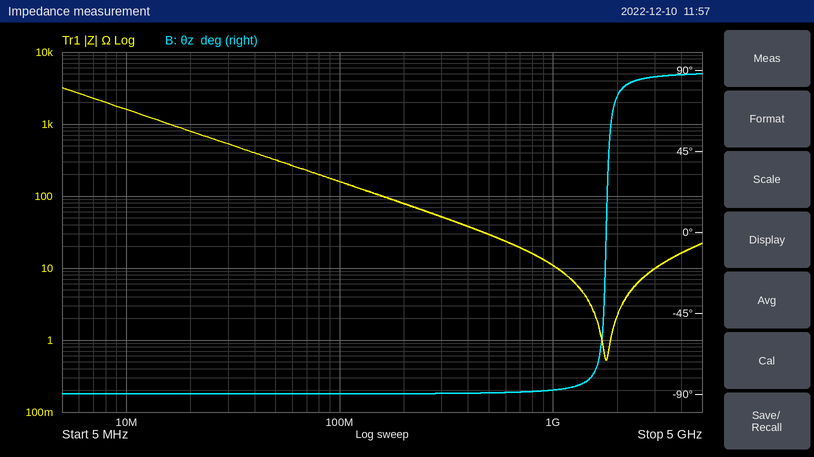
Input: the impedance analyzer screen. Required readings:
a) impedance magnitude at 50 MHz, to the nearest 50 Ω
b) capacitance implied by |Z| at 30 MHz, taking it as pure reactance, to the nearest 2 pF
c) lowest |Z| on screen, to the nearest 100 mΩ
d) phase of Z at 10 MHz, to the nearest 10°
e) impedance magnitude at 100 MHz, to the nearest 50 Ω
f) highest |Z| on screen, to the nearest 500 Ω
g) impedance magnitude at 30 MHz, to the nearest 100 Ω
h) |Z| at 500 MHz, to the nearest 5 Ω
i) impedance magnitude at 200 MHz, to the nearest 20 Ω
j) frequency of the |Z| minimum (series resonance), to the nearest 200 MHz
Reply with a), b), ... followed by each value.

a) 300 Ω
b) 10 pF
c) 500 mΩ
d) -90°
e) 150 Ω
f) 3.0 kΩ
g) 500 Ω
h) 30 Ω
i) 80 Ω
j) 1.8 GHz
